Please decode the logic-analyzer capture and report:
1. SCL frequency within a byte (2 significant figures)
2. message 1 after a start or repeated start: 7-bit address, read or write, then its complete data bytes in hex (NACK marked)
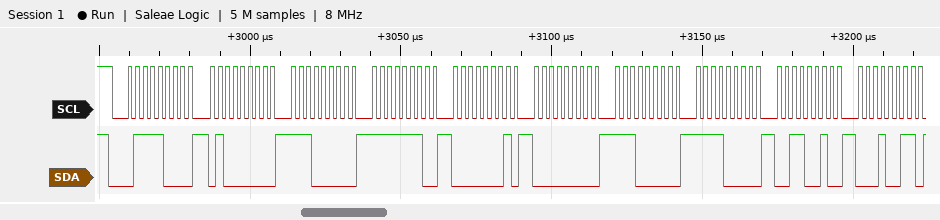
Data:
400 kHz
0x3C write: 40 E0 FE 01 00 E0 F0 32 13
